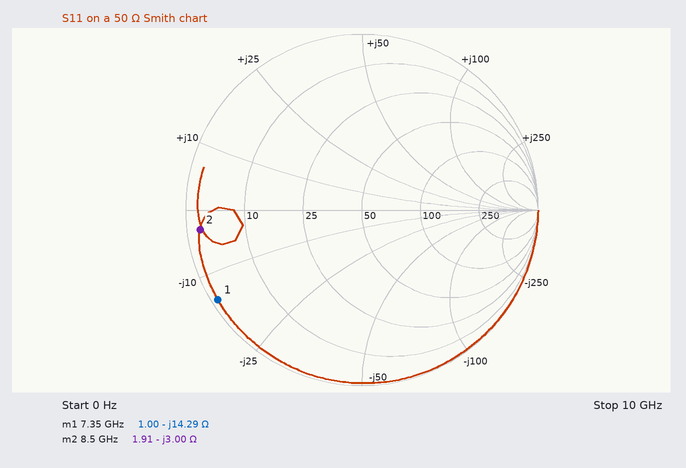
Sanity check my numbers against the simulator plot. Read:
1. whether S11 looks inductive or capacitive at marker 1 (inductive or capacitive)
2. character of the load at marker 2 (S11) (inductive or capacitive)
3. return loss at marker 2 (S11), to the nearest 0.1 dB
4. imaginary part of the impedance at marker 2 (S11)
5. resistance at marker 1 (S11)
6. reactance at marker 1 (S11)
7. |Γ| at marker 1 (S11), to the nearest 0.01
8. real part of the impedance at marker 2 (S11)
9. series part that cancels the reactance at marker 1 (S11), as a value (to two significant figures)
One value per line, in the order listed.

capacitive
capacitive
0.7 dB
-3.00 Ω
1.00 Ω
-14.29 Ω
0.96
1.91 Ω
310 pH
